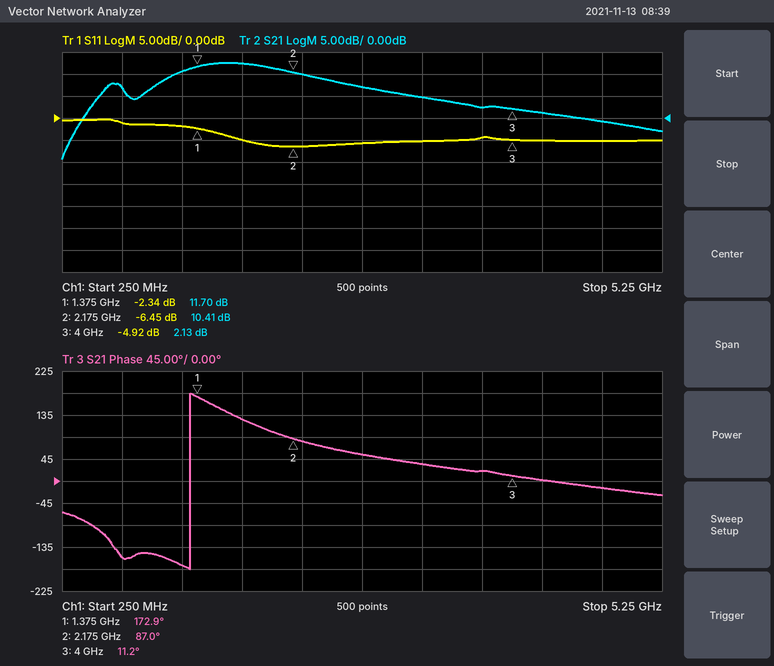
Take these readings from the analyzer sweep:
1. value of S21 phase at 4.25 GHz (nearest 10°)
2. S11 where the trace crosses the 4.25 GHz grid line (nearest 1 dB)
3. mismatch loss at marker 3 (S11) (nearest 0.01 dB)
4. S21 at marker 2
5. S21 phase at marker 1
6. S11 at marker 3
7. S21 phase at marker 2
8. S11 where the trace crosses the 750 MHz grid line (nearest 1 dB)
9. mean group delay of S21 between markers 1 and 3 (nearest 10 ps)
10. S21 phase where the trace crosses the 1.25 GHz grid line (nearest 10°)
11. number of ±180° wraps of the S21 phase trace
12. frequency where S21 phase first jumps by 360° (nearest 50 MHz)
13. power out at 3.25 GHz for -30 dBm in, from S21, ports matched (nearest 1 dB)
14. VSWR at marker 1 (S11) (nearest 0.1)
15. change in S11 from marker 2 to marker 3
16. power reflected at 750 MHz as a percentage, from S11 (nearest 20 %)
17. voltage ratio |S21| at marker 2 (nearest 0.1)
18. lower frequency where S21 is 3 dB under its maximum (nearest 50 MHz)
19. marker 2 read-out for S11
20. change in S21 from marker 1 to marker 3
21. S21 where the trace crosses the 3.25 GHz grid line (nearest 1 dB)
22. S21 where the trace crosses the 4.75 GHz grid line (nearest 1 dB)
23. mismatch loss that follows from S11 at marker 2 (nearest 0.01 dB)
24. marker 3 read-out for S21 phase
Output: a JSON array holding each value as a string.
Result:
["0°", "-5 dB", "1.69 dB", "10.41 dB", "172.9°", "-4.92 dB", "87.0°", "-1 dB", "170 ps", "-170°", "1", "1.30 GHz", "-25 dBm", "7.5", "1.53 dB", "80 %", "3.3", "1.15 GHz", "-6.45 dB", "-9.57 dB", "5 dB", "-1 dB", "1.12 dB", "11.2°"]
